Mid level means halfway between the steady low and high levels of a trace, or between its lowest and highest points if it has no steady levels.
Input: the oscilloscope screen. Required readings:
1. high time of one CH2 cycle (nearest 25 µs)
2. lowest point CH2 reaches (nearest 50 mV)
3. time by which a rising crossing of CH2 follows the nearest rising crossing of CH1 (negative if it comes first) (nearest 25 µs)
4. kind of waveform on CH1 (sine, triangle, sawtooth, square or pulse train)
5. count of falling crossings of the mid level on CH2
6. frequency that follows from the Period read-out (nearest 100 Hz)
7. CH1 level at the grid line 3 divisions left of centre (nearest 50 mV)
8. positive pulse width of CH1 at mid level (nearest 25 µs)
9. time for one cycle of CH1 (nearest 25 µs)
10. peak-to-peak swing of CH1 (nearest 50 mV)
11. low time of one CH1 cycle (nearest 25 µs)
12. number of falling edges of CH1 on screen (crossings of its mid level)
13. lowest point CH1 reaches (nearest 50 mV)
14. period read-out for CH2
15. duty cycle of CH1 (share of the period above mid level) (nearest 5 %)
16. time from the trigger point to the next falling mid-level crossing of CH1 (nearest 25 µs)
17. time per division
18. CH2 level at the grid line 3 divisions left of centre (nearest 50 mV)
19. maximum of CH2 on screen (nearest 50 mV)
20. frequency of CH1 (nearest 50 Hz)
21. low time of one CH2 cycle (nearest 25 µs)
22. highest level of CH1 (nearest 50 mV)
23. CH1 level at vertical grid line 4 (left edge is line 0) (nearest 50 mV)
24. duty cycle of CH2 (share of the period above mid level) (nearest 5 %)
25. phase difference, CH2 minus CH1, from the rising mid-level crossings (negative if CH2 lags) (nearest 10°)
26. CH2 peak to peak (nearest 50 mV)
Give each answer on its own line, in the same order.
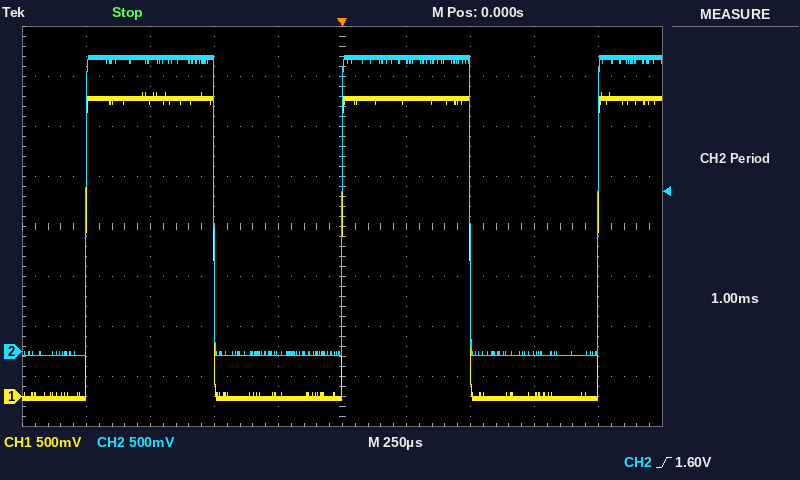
500 µs
-50 mV
0 µs
square
2
1.0 kHz
2.95 V
500 µs
1.000 ms
3.10 V
500 µs
2
-50 mV
1.00 ms
50 %
500 µs
250 µs
2.90 V
2.95 V
1.00 kHz
500 µs
3.05 V
0 mV
50 %
0°
3.00 V
